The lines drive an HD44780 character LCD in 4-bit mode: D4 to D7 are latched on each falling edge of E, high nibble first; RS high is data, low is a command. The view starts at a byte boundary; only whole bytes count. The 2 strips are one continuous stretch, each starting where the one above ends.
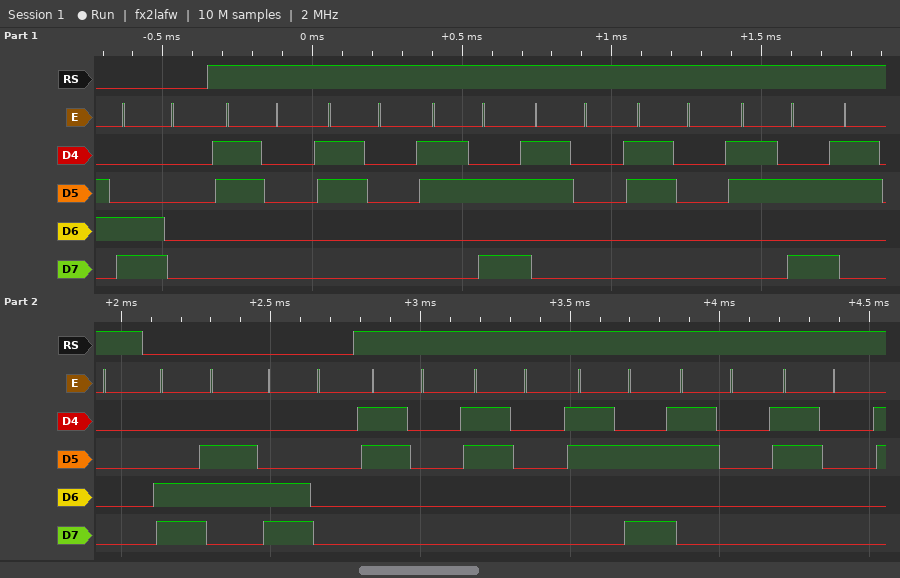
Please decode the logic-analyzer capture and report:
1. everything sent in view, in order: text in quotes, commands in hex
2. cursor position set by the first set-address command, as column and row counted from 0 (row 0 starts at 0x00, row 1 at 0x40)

0xC0 "00:00:0" 0xC6 0xC0 "00:00"
column 0, row 1
